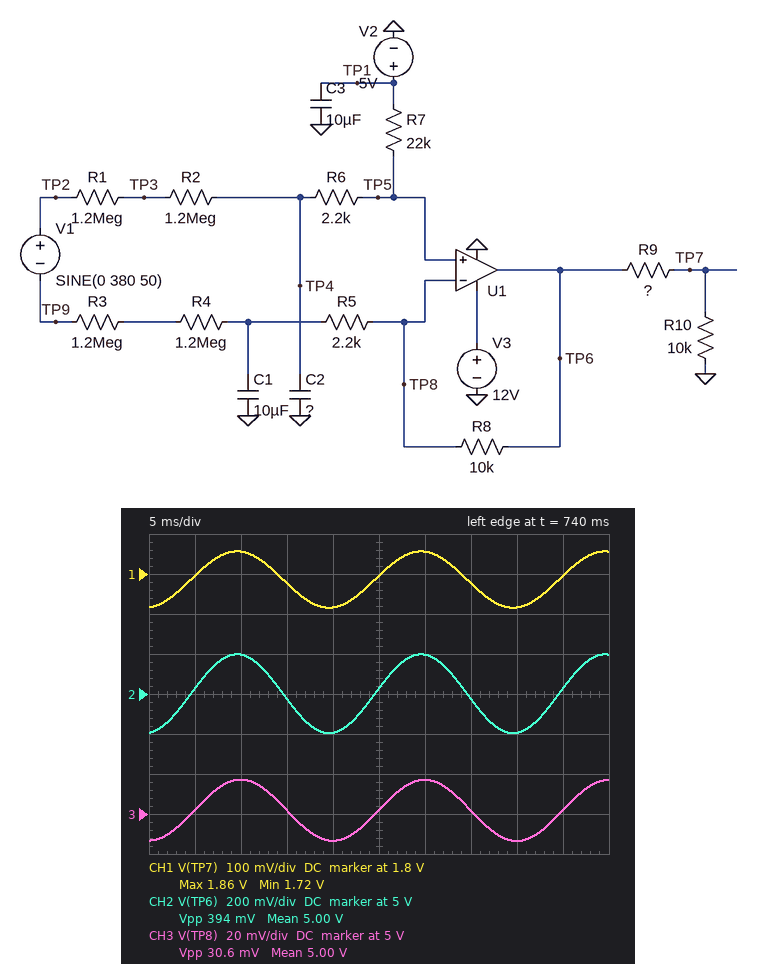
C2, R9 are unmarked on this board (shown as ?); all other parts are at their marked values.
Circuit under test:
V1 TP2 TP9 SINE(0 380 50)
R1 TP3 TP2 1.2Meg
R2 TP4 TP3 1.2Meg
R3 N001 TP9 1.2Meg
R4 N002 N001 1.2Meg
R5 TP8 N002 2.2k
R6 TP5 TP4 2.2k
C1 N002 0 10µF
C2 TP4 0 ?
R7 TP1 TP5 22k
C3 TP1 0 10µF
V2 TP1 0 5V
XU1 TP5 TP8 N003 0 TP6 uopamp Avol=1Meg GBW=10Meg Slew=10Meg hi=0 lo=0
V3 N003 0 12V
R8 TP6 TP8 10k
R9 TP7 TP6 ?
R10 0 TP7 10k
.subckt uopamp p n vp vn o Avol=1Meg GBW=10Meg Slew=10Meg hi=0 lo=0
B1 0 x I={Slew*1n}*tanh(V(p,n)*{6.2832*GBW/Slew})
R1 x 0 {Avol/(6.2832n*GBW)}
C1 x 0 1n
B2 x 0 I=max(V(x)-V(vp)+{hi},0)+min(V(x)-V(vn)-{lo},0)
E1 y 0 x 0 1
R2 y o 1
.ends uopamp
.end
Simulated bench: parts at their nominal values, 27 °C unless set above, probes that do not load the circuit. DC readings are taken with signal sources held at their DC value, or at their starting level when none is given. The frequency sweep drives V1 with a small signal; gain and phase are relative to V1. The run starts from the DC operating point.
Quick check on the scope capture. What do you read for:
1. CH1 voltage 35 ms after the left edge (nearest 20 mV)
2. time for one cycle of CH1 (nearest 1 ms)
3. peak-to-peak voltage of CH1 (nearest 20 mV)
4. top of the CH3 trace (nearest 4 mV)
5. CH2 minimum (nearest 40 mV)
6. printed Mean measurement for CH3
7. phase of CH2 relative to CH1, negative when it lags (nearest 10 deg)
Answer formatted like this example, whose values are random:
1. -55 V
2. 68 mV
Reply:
1. 1.78 V
2. 20 ms
3. 140 mV
4. 5.016 V
5. 4.80 V
6. 5.00 V
7. 0 deg
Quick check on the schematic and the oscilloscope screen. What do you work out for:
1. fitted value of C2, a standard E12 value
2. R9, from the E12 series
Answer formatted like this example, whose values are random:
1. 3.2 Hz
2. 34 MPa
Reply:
1. 15 µF
2. 18 kΩ
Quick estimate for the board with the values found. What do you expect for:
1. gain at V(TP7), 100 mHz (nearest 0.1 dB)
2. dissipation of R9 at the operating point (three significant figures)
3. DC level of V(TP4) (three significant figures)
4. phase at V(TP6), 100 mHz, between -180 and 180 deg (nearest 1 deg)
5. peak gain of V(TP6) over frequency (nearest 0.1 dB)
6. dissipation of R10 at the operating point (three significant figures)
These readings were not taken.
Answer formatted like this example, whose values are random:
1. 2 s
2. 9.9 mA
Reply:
1. -52.6 dB
2. 574 µW
3. 5.00 V
4. -7 deg
5. -43.5 dB
6. 319 µW
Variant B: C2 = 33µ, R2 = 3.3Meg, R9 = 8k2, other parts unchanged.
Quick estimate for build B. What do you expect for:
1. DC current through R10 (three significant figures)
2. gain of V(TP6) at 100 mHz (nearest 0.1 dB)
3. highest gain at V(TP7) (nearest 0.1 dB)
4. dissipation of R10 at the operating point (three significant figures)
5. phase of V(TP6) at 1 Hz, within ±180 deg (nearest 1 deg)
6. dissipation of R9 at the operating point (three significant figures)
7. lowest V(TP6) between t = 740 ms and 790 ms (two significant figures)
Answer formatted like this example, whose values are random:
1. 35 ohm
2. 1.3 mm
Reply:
1. 275 µA
2. -47.5 dB
3. -51.9 dB
4. 755 µW
5. -22 deg
6. 619 µW
7. 4.9 V
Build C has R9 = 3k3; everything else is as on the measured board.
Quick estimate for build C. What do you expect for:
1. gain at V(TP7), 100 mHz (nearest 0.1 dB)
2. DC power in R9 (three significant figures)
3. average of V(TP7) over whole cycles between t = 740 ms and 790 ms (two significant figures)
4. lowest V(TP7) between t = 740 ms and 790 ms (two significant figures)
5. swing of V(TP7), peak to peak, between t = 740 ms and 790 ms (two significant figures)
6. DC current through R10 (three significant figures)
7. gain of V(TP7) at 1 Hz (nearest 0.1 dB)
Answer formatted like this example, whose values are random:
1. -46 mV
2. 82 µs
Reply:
1. -46.2 dB
2. 466 µW
3. 3.8 V
4. 3.6 V
5. 300 mV
6. 376 µA
7. -50.0 dB
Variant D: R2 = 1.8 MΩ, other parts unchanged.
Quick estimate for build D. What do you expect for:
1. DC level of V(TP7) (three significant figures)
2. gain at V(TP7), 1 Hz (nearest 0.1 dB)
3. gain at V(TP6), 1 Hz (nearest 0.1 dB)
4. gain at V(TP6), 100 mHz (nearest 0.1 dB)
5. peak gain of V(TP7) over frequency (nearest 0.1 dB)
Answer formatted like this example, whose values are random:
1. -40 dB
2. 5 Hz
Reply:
1. 1.79 V
2. -57.5 dB
3. -48.5 dB
4. -44.7 dB
5. -53.5 dB
